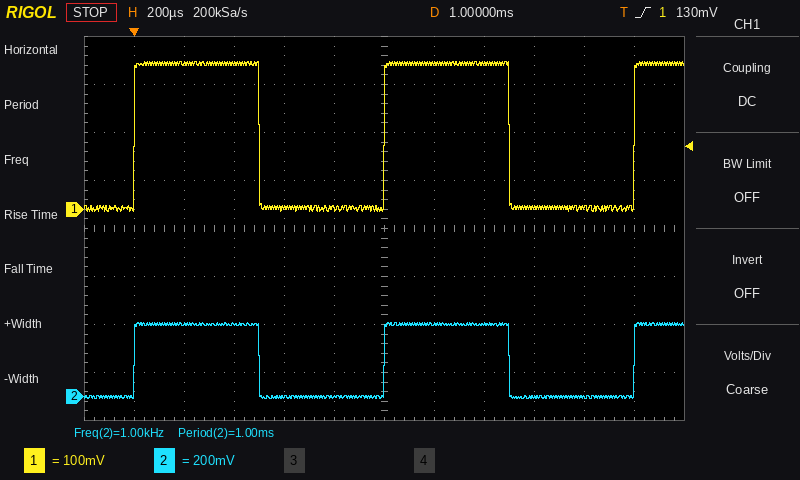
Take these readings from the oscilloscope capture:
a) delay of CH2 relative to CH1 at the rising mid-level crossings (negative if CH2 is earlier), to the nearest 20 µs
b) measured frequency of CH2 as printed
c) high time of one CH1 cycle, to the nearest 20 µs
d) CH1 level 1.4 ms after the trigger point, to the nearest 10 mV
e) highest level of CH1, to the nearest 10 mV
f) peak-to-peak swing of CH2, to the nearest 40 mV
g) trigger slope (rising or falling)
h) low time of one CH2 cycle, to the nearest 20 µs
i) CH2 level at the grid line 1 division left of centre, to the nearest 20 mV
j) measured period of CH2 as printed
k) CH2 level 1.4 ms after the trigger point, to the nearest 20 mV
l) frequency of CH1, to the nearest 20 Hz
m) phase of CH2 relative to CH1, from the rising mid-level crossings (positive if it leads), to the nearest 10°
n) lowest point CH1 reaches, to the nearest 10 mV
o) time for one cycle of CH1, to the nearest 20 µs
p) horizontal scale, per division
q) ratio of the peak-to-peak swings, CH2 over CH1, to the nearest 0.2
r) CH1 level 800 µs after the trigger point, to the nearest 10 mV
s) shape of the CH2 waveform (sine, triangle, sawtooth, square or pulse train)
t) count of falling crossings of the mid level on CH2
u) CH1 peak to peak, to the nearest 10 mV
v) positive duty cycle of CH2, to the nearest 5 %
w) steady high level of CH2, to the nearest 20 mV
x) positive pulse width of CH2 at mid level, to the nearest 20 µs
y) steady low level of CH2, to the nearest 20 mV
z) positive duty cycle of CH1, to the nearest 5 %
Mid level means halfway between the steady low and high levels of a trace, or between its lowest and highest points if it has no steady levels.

0 µs
1.00 kHz
500 µs
300 mV
310 mV
320 mV
rising
500 µs
0 mV
1.00 ms
300 mV
1.00 kHz
0°
0 mV
1.00 ms
200 µs
1.0
0 mV
square
2
310 mV
50 %
300 mV
500 µs
0 mV
50 %
